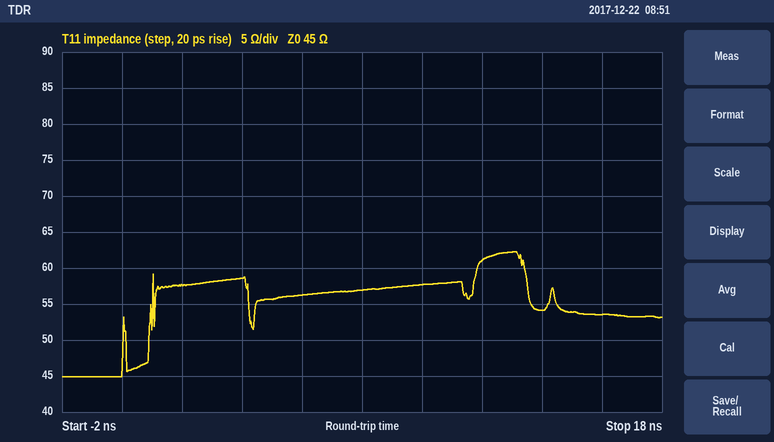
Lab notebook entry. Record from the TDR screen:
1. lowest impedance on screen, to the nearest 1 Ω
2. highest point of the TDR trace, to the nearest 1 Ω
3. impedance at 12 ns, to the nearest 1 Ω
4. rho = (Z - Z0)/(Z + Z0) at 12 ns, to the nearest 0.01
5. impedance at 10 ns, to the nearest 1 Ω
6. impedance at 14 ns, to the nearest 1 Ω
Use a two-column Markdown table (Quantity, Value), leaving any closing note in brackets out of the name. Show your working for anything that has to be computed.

| Quantity | Value |
|---|---|
| lowest impedance on screen, to the nearest 1 Ω | 45 Ω |
| highest point of the TDR trace, to the nearest 1 Ω | 62 Ω |
| impedance at 12 ns, to the nearest 1 Ω | 61 Ω |
| rho = (Z - Z0)/(Z + Z0) at 12 ns, to the nearest 0.01 | (61 − 45)/(61 + 45) ≈ +0.15 |
| impedance at 10 ns, to the nearest 1 Ω | 58 Ω |
| impedance at 14 ns, to the nearest 1 Ω | 54 Ω |
